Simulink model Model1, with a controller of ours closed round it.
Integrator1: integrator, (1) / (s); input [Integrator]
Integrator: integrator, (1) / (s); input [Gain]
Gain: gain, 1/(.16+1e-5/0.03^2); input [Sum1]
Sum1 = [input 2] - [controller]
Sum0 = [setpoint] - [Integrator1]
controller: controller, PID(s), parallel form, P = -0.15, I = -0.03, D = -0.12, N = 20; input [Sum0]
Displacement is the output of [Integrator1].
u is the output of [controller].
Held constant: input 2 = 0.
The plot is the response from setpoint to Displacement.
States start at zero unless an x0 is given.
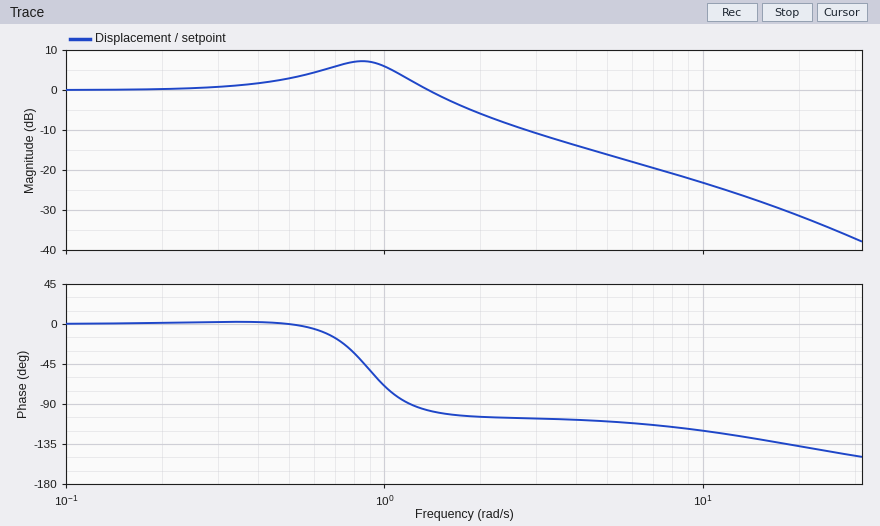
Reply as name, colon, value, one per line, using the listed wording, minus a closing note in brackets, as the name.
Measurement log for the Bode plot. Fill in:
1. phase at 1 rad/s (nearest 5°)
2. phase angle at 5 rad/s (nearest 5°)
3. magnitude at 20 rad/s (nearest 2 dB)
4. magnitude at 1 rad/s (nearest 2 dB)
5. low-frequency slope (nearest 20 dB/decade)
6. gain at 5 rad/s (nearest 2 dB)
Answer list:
phase at 1 rad/s: -70°
phase angle at 5 rad/s: -110°
magnitude at 20 rad/s: -32 dB
magnitude at 1 rad/s: 6 dB
low-frequency slope: 0 dB/decade
gain at 5 rad/s: -16 dB
